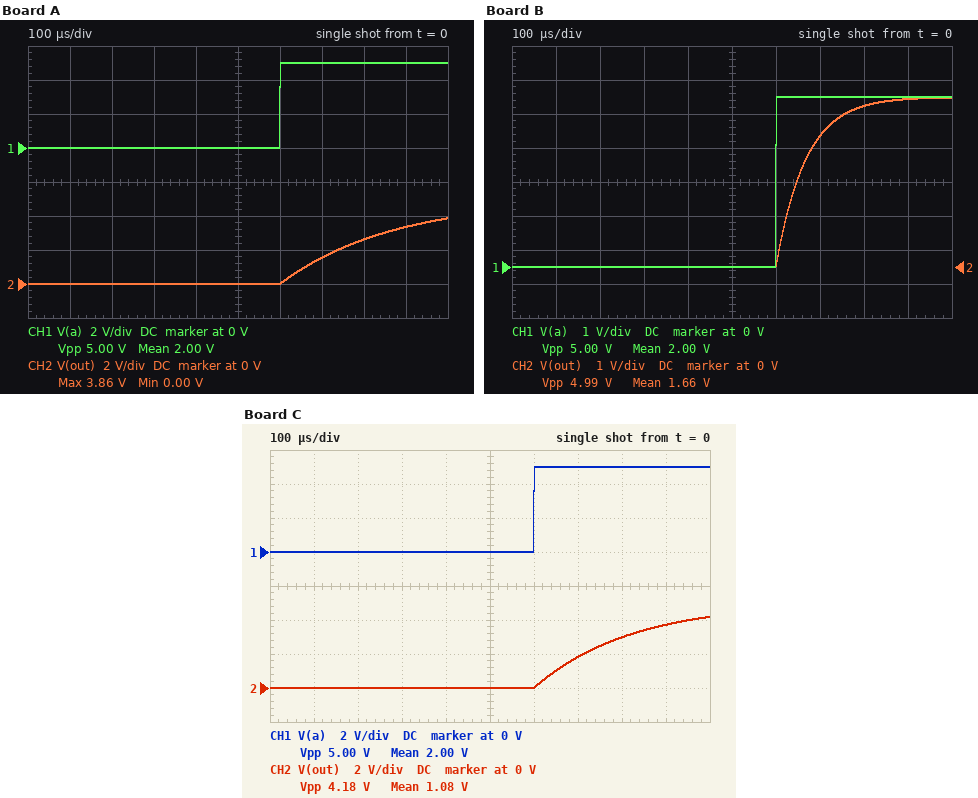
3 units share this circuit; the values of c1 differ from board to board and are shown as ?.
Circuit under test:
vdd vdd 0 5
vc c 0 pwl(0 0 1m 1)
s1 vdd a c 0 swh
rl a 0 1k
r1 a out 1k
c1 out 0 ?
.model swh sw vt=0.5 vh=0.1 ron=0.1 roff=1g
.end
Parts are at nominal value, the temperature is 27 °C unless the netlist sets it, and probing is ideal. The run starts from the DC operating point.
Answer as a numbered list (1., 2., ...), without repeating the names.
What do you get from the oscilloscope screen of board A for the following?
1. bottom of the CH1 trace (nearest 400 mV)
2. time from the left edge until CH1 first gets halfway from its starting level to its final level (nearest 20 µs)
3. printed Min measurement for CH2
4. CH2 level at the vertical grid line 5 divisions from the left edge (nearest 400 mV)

1. 0 V
2. 600 µs
3. 0.00 V
4. 0 V
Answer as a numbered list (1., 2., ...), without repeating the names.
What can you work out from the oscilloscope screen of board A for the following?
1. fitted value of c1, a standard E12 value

1. 270 nF
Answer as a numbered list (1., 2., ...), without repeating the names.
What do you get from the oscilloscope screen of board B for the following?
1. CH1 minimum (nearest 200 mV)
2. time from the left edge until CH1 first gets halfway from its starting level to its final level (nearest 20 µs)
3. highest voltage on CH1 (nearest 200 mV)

1. 0 V
2. 600 µs
3. 5.0 V
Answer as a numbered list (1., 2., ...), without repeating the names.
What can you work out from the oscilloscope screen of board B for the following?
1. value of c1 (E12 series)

1. 68 nF
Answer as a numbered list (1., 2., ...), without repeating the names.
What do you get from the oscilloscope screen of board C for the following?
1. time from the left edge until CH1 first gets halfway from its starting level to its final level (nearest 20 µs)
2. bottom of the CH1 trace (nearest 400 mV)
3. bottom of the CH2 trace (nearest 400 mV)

1. 600 µs
2. 0 V
3. 0 V
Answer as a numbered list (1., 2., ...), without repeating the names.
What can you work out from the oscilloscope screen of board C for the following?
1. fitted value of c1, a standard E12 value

1. 220 nF
